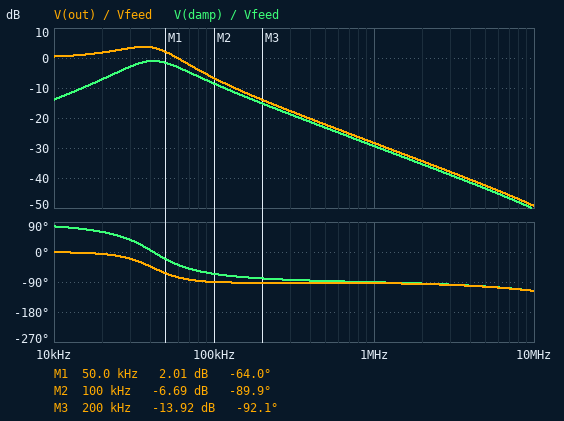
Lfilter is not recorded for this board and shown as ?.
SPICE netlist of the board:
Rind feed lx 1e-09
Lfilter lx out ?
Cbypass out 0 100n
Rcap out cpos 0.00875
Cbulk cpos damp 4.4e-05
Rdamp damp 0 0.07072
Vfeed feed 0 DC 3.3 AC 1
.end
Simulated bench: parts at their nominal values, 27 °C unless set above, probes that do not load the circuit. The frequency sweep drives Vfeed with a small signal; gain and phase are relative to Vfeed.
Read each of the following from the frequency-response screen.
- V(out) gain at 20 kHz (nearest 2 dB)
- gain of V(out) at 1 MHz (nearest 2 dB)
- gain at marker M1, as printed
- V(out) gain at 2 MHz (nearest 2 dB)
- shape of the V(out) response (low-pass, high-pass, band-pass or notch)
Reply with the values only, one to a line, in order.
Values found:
2 dB
-28 dB
2.01 dB
-34 dB
low-pass
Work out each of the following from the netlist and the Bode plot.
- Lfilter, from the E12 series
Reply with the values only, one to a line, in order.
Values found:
330 nH
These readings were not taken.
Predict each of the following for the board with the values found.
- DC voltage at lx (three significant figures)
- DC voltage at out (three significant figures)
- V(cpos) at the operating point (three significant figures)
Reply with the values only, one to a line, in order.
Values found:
3.30 V
3.30 V
3.30 V
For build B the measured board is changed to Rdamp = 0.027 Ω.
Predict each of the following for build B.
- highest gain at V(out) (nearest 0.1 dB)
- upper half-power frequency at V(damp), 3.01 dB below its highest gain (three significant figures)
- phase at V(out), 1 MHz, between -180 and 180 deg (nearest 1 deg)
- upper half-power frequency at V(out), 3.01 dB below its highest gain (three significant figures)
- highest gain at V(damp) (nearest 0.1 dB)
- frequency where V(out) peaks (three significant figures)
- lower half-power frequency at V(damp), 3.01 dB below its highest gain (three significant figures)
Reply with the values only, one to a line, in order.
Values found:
8.5 dB
51.2 kHz
-96 deg
48.3 kHz
-2.4 dB
40.2 kHz
34.0 kHz
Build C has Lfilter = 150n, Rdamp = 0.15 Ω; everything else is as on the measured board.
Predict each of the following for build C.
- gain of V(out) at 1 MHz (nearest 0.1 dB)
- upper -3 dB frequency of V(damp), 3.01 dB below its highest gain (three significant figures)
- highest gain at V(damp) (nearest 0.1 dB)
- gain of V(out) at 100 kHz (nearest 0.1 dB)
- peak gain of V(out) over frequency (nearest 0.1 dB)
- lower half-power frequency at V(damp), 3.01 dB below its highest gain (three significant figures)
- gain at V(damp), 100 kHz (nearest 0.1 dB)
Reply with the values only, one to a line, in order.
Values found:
-15.5 dB
191 kHz
-0.5 dB
-0.3 dB
0.8 dB
20.4 kHz
-1.0 dB
